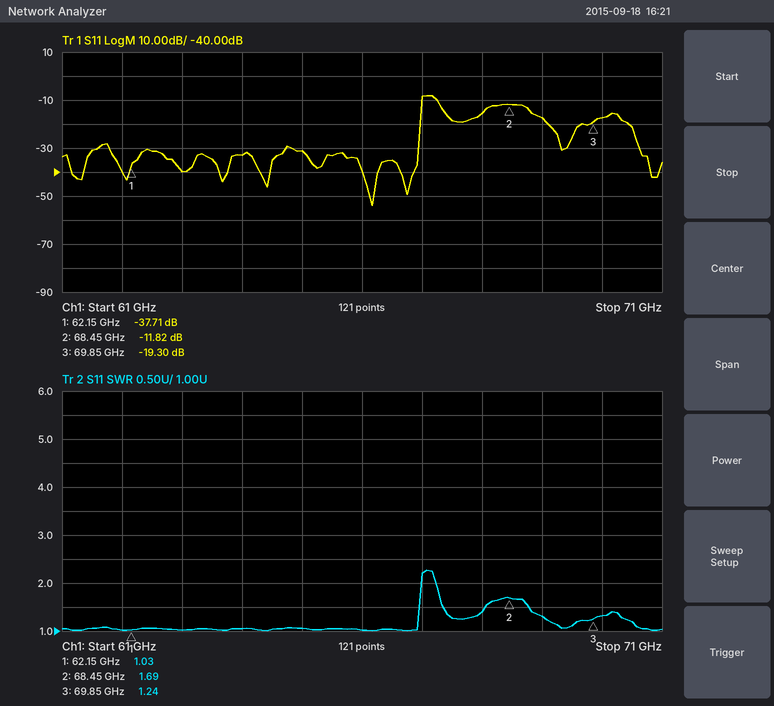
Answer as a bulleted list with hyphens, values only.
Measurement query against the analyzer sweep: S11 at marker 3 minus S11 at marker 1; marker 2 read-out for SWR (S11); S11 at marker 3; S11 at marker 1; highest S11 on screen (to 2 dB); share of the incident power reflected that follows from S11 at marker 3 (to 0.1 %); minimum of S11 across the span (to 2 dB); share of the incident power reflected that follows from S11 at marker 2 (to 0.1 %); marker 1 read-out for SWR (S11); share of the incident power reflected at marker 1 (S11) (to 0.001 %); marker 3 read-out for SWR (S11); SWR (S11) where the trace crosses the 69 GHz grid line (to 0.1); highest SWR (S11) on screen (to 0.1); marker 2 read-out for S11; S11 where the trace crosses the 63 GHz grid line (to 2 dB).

- 18.41 dB
- 1.69
- -19.30 dB
- -37.71 dB
- -8 dB
- 1.2 %
- -54 dB
- 6.6 %
- 1.03
- 0.017 %
- 1.24
- 1.3
- 2.3
- -11.82 dB
- -40 dB
